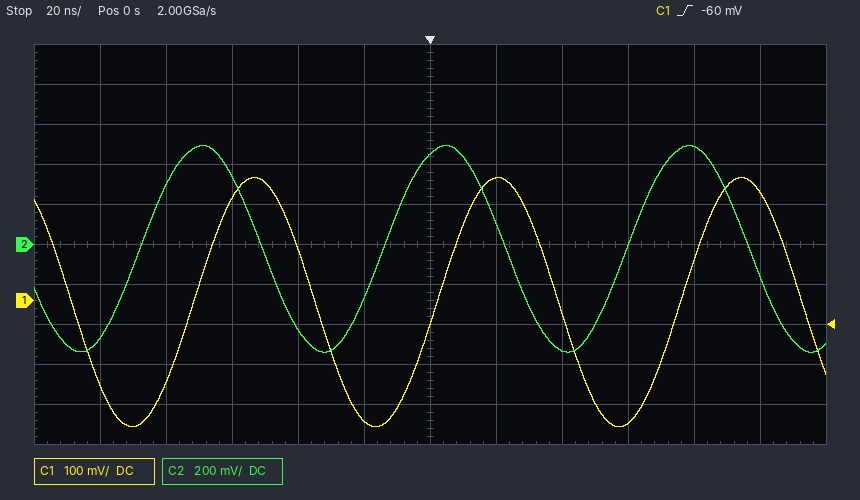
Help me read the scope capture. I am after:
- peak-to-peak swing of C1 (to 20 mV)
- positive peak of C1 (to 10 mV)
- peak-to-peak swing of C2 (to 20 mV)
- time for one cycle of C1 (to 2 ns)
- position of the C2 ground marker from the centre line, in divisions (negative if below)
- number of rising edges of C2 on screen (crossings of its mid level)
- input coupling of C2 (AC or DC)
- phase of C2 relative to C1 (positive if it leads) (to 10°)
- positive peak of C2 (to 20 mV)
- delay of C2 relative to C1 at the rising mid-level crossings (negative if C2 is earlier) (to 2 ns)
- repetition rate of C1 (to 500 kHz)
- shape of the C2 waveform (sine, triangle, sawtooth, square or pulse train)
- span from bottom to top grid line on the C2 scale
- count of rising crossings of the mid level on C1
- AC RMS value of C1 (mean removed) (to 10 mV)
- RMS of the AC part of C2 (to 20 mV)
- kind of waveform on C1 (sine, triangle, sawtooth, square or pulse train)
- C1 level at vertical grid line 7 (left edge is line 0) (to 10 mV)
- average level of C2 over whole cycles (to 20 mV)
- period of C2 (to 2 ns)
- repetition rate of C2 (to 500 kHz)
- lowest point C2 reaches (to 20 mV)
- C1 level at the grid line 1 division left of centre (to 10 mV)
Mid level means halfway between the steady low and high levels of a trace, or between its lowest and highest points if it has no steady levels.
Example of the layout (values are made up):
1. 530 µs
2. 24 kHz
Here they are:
1. 620 mV
2. 310 mV
3. 1.04 V
4. 74 ns
5. 0.0 div
6. 3
7. DC
8. +80°
9. 500 mV
10. -16 ns
11. 13.5 MHz
12. sine
13. 2 V
14. 3
15. 220 mV
16. 360 mV
17. sine
18. 310 mV
19. -20 mV
20. 74 ns
21. 13.5 MHz
22. -540 mV
23. -300 mV
